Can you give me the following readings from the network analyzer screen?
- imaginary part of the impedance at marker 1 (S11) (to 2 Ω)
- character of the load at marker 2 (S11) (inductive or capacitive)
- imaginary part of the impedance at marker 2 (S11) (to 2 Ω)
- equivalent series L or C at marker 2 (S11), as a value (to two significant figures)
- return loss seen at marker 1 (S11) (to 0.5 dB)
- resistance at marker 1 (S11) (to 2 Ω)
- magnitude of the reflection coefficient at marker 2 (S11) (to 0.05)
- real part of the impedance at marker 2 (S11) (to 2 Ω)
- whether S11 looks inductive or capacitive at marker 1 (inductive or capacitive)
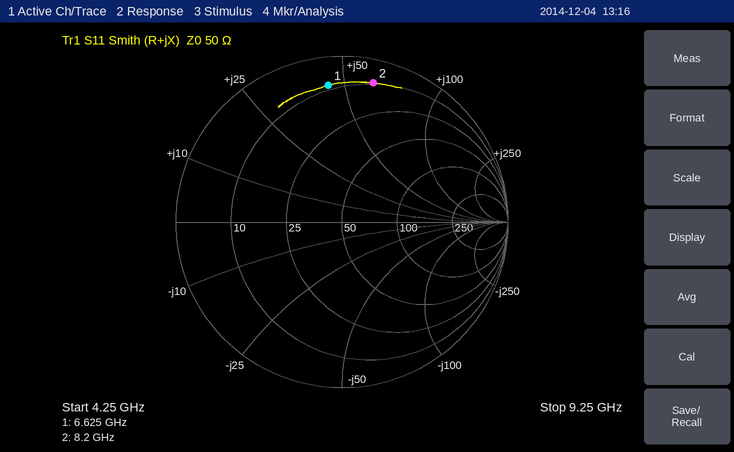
+44 Ω
inductive
+62 Ω
1.2 nH
1.5 dB
8 Ω
0.85
10 Ω
inductive
